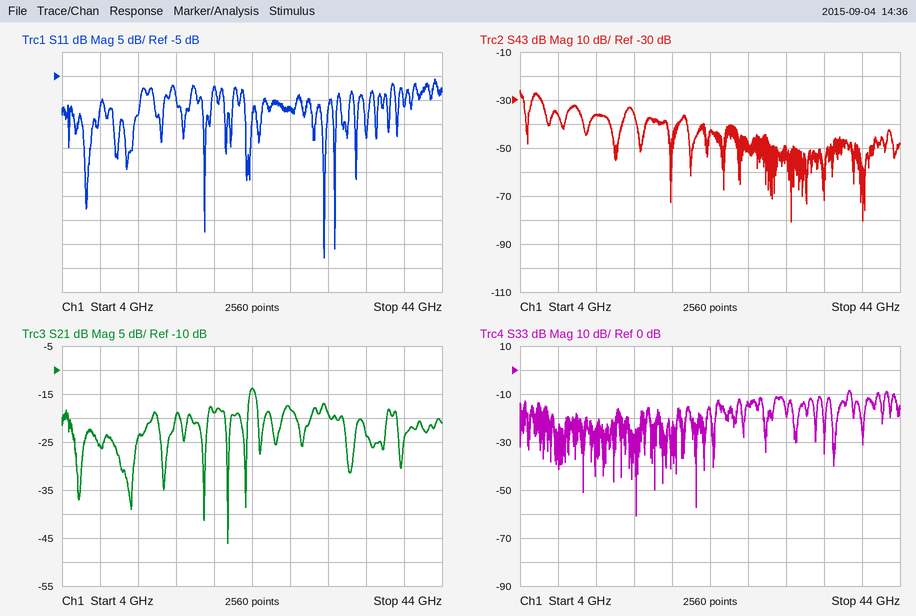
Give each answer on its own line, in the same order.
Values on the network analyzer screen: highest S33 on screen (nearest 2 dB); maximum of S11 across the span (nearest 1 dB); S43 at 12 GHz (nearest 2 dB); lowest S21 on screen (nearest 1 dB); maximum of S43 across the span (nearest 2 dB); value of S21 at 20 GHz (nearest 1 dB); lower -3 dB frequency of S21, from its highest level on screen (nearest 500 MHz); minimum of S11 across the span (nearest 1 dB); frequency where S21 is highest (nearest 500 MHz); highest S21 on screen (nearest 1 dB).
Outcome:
-8 dB
-6 dB
-36 dB
-46 dB
-26 dB
-19 dB
23.5 GHz
-43 dB
24.0 GHz
-14 dB
